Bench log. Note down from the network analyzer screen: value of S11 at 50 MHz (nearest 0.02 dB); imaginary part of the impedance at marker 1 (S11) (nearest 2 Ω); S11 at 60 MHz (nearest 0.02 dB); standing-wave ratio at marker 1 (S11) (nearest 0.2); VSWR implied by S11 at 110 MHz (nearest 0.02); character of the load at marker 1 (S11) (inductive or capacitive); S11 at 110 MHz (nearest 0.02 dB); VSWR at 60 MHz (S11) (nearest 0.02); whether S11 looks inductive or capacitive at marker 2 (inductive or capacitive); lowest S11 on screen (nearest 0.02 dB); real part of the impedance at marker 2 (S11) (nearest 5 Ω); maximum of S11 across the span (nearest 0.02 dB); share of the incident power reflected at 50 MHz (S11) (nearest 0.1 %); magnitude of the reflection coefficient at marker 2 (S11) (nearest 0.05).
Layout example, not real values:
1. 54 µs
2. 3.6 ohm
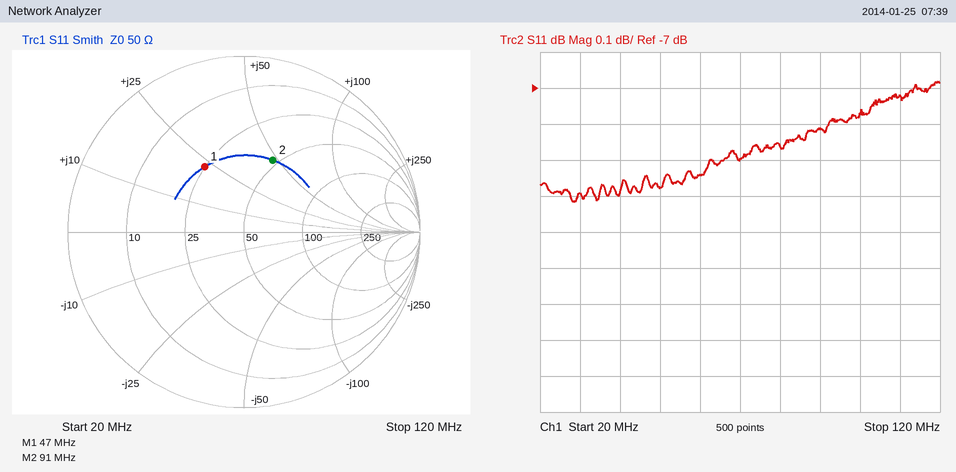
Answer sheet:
1. -7.28 dB
2. +22 Ω
3. -7.24 dB
4. 2.6
5. 2.60
6. inductive
7. -7.02 dB
8. 2.54
9. inductive
10. -7.32 dB
11. 45 Ω
12. -6.98 dB
13. 18.7 %
14. 0.45
